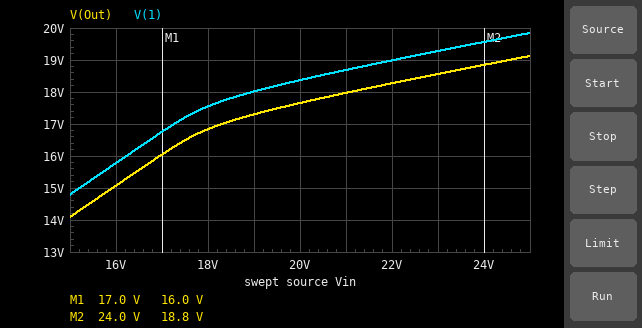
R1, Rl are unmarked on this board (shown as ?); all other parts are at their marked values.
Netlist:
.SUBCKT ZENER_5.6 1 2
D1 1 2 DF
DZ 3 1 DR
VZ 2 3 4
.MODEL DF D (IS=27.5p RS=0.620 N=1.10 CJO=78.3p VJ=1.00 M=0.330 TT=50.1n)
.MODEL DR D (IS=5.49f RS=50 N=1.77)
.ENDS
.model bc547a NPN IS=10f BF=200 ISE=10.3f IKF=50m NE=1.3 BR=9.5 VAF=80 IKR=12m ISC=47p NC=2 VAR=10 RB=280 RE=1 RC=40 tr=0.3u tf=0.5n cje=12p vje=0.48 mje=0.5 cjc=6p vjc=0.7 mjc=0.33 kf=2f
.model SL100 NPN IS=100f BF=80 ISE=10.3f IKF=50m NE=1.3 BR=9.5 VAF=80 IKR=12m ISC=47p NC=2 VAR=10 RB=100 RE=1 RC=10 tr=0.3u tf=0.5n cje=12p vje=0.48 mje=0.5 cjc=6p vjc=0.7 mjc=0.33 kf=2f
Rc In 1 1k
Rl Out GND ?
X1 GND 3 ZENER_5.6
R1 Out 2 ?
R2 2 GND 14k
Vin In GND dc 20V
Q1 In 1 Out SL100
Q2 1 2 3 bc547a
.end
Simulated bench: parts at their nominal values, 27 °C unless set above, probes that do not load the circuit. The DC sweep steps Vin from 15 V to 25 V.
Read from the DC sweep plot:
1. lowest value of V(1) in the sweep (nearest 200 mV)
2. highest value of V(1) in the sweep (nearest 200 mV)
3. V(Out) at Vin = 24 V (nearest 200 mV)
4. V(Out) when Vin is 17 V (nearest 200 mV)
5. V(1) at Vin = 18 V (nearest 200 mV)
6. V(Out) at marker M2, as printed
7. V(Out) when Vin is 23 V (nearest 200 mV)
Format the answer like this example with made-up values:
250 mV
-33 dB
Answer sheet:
14.8 V
19.8 V
18.8 V
16.0 V
17.6 V
18.8 V
18.6 V
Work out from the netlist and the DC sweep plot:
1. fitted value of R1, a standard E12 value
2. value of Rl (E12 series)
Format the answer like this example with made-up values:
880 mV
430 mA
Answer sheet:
27 kΩ
1.2 kΩ
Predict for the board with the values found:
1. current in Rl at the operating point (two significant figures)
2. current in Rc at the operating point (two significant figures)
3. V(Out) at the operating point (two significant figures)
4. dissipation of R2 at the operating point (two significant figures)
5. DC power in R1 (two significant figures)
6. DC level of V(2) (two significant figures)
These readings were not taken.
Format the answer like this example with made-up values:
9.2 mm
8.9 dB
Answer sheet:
15 mA
1.6 mA
18 V
2.5 mW
5.1 mW
5.9 V
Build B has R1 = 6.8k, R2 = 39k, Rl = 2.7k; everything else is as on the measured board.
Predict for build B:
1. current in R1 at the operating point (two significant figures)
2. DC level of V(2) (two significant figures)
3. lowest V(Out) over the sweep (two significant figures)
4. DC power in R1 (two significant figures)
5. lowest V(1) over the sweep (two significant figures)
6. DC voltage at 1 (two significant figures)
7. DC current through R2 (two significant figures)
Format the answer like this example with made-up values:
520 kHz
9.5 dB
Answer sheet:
260 µA
6.6 V
7.8 V
470 µW
8.4 V
9.0 V
170 µA
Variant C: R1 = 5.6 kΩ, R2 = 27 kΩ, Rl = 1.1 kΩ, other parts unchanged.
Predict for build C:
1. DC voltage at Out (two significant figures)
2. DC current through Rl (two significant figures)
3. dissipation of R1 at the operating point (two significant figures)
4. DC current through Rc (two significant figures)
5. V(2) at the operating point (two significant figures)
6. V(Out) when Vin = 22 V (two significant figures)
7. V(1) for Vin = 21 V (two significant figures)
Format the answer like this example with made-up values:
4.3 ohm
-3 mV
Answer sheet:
8.5 V
7.7 mA
630 µW
11 mA
6.6 V
8.7 V
9.3 V
